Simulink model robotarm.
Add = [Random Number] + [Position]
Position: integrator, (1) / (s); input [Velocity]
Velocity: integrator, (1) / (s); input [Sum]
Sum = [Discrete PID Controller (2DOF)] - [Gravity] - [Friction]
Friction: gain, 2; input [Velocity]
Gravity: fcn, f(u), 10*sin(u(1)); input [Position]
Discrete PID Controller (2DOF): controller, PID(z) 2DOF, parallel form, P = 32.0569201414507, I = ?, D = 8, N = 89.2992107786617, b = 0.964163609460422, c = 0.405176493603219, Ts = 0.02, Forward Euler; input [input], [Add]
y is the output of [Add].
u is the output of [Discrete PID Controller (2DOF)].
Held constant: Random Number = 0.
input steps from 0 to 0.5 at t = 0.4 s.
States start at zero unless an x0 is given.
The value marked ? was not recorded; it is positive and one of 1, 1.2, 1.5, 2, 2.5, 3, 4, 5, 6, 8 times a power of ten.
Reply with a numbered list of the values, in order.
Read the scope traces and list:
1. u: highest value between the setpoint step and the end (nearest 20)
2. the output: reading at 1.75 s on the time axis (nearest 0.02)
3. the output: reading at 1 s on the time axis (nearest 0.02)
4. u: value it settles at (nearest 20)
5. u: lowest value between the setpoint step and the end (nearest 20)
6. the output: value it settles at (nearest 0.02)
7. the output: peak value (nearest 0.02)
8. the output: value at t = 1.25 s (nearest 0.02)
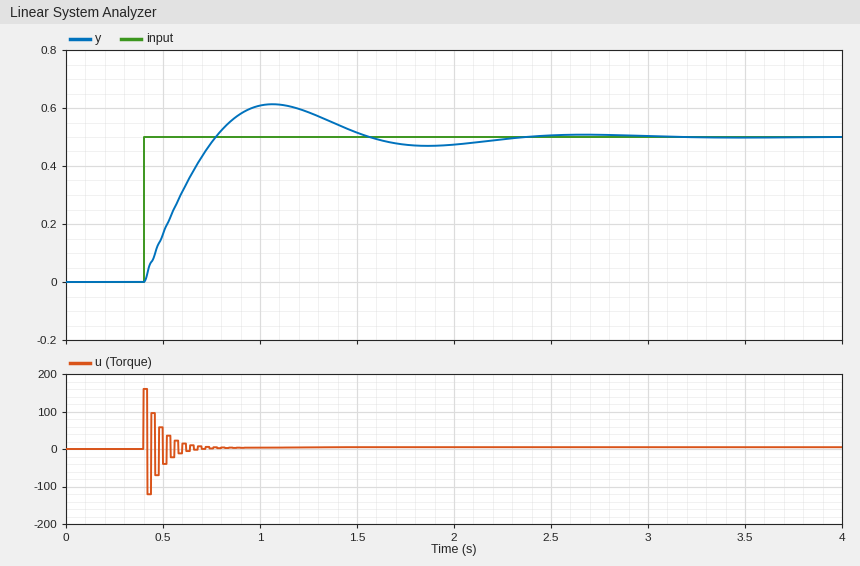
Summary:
1. 160
2. 0.48
3. 0.60
4. 0
5. -120
6. 0.50
7. 0.62
8. 0.58
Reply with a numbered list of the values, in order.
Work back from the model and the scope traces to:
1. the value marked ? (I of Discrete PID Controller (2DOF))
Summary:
1. 120
